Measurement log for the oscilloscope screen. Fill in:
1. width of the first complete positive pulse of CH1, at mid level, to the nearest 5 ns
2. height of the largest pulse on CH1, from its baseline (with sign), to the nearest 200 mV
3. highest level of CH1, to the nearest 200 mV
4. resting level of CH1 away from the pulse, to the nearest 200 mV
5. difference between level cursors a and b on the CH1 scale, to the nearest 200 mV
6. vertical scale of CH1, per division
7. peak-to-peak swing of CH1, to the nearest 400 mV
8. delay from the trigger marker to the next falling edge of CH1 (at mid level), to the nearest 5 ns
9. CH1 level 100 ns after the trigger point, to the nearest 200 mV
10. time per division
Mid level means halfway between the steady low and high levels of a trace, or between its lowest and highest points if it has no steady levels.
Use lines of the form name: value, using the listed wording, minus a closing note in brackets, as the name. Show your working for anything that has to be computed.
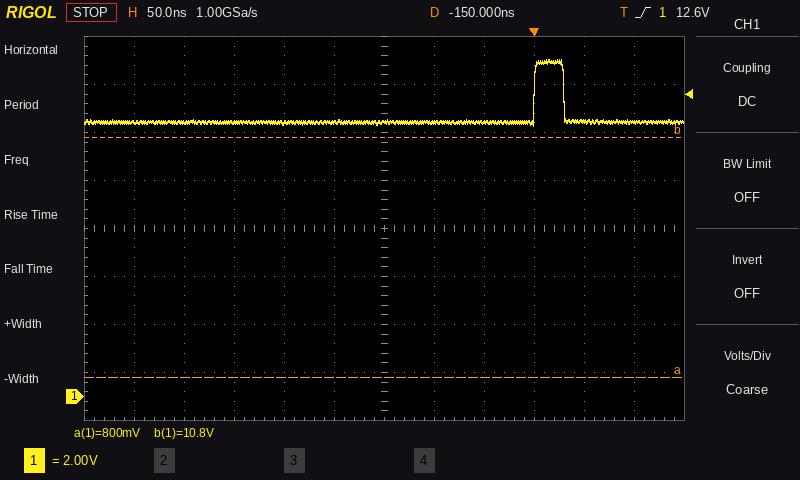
width of the first complete positive pulse of CH1, at mid level, to the nearest 5 ns: 30 ns
height of the largest pulse on CH1, from its baseline (with sign), to the nearest 200 mV: 14.0 V − (11.4 V) = +2.6 V
highest level of CH1, to the nearest 200 mV: 14.0 V
resting level of CH1 away from the pulse, to the nearest 200 mV: 11.4 V
difference between level cursors a and b on the CH1 scale, to the nearest 200 mV: 10.0 V
vertical scale of CH1, per division: 2 V
peak-to-peak swing of CH1, to the nearest 400 mV: 2.8 V
delay from the trigger marker to the next falling edge of CH1 (at mid level), to the nearest 5 ns: 30 ns
CH1 level 100 ns after the trigger point, to the nearest 200 mV: 11.4 V
time per division: 50 ns
